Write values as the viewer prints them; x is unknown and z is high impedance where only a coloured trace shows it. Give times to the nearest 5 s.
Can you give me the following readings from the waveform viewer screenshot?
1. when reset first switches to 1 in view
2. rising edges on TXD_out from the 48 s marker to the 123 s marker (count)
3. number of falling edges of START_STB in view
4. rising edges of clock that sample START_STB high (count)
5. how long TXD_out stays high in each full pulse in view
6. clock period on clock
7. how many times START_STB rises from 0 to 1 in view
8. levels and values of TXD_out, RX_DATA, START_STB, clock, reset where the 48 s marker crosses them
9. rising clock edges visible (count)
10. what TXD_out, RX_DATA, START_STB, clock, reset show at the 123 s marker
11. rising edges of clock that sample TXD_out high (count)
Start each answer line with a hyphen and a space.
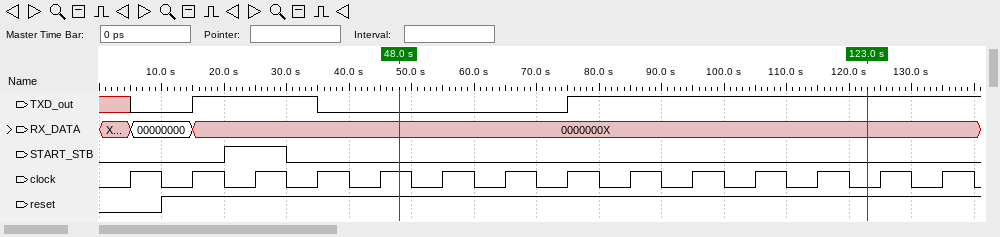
- 10 s
- 1
- 1
- 1
- 20 s
- 10 s
- 1
- TXD_out=0, RX_DATA=0000000X, START_STB=0, clock=1, reset=1
- 14
- TXD_out=1, RX_DATA=0000000X, START_STB=0, clock=0, reset=1
- 8
